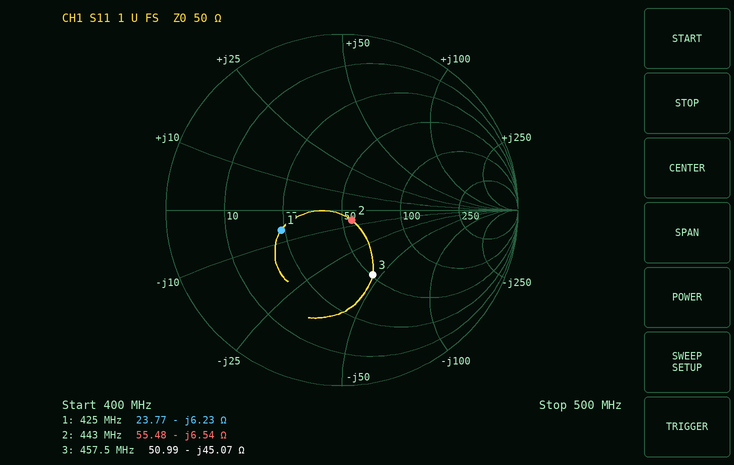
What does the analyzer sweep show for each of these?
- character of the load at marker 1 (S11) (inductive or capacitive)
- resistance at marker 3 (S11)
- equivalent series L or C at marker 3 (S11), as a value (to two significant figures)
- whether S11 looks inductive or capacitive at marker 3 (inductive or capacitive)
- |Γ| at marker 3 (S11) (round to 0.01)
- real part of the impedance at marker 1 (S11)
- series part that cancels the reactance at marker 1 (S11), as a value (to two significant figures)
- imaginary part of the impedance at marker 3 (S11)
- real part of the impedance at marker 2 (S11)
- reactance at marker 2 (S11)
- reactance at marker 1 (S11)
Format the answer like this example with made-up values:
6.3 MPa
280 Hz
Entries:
capacitive
50.99 Ω
7.7 pF
capacitive
0.41
23.77 Ω
2.3 nH
-45.07 Ω
55.48 Ω
-6.54 Ω
-6.23 Ω
